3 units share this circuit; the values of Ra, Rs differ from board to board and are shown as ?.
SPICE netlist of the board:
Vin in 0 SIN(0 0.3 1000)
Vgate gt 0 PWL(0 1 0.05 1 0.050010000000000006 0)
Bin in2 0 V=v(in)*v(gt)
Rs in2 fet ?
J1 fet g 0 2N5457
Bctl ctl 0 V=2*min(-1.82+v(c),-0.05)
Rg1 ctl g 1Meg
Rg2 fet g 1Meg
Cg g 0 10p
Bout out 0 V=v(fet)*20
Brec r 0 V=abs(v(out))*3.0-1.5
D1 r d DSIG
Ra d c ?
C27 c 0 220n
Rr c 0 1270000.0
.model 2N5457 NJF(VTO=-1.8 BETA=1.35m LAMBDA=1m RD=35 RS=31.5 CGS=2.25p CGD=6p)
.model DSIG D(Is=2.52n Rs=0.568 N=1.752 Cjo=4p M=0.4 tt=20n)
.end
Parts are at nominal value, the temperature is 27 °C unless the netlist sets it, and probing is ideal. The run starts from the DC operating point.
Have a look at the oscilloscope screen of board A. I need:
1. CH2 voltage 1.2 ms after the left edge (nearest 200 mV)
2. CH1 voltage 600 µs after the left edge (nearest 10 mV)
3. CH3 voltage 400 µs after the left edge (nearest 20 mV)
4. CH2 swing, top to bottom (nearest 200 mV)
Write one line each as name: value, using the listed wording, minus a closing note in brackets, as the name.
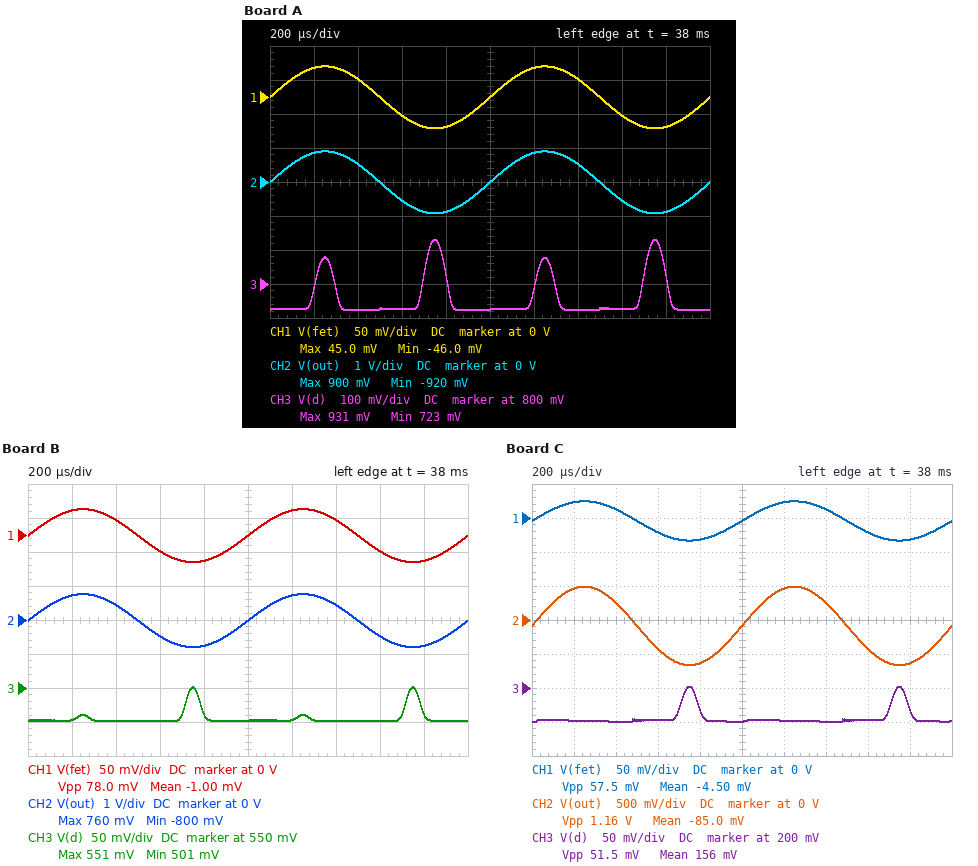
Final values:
CH2 voltage 1.2 ms after the left edge: 800 mV
CH1 voltage 600 µs after the left edge: -30 mV
CH3 voltage 400 µs after the left edge: 720 mV
CH2 swing, top to bottom: 1.8 V
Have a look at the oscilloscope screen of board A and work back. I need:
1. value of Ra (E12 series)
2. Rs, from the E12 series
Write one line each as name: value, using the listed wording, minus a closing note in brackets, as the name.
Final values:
value of Ra: 47 kΩ
Rs, from the E12 series: 3.3 kΩ
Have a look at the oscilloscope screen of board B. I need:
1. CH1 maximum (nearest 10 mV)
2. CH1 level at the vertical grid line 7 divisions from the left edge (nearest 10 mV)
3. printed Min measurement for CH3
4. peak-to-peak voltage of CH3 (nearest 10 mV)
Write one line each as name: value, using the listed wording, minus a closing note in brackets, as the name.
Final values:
CH1 maximum: 40 mV
CH1 level at the vertical grid line 7 divisions from the left edge: 20 mV
printed Min measurement for CH3: 501 mV
peak-to-peak voltage of CH3: 50 mV
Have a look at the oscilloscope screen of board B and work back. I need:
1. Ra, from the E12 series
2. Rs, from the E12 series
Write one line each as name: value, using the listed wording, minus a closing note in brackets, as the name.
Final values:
Ra, from the E12 series: 10 kΩ
Rs, from the E12 series: 5.6 kΩ
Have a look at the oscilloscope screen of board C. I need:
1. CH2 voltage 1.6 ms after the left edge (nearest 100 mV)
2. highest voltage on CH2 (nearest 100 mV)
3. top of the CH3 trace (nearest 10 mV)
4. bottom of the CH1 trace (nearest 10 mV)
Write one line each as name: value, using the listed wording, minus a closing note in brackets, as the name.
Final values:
CH2 voltage 1.6 ms after the left edge: -400 mV
highest voltage on CH2: 500 mV
top of the CH3 trace: 200 mV
bottom of the CH1 trace: -30 mV
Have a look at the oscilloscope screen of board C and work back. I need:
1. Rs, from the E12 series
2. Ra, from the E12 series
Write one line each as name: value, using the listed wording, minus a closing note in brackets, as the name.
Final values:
Rs, from the E12 series: 27 kΩ
Ra, from the E12 series: 33 kΩ
